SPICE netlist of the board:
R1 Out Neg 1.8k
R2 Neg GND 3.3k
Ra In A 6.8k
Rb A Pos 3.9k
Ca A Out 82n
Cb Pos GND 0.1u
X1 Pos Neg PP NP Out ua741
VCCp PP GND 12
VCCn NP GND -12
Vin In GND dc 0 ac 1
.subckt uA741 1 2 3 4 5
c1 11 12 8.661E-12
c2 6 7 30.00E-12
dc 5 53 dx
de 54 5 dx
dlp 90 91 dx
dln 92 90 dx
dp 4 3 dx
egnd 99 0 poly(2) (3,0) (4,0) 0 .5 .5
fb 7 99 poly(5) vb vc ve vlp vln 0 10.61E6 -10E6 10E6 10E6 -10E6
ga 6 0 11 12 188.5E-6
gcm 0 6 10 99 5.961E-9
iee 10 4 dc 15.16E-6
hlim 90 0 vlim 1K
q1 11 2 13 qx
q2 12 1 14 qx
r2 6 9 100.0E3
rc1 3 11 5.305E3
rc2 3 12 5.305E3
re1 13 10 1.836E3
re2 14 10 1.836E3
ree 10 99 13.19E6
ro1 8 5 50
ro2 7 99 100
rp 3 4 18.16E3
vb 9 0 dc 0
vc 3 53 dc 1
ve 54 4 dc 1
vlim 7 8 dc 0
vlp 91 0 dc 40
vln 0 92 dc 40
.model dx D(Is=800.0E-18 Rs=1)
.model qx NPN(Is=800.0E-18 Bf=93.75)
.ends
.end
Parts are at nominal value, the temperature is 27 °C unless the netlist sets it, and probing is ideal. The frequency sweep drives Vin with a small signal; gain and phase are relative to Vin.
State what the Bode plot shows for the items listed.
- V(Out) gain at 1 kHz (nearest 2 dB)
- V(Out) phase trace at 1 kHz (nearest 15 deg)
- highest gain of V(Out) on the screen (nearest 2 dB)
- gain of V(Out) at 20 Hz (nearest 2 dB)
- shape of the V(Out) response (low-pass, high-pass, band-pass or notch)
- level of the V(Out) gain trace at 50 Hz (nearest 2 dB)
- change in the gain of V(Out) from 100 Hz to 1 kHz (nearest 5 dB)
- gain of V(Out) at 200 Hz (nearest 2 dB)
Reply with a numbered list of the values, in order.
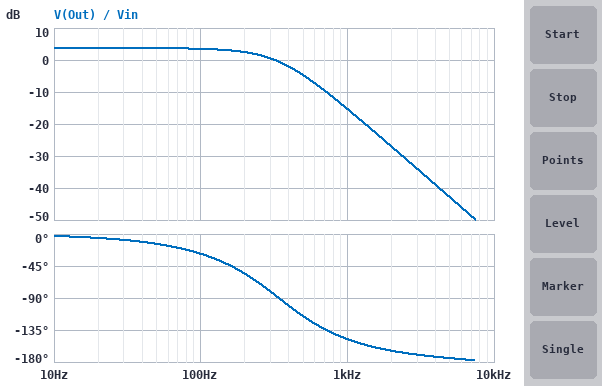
1. -16 dB
2. -150 deg
3. 4 dB
4. 4 dB
5. low-pass
6. 4 dB
7. -20 dB
8. 2 dB
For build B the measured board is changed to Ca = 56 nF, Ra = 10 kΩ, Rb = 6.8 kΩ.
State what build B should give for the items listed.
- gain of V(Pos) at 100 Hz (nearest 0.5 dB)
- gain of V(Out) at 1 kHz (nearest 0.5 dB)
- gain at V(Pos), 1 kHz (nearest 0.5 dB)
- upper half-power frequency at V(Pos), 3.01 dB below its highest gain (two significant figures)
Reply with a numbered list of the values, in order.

1. -1.5 dB
2. -20.5 dB
3. -24.5 dB
4. 140 Hz
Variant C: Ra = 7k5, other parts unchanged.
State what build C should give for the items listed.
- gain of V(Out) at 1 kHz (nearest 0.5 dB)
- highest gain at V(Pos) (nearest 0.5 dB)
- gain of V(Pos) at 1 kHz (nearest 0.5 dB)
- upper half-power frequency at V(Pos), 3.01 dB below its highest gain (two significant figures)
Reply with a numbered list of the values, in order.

1. -16.0 dB
2. 0 dB
3. -20.0 dB
4. 270 Hz
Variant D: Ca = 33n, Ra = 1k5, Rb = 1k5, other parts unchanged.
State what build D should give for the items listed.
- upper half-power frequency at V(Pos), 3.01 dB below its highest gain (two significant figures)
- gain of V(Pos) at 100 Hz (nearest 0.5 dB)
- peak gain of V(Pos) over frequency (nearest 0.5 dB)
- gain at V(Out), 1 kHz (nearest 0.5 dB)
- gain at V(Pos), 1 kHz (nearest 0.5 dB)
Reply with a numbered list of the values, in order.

1. 650 Hz
2. 0 dB
3. 0 dB
4. -1.5 dB
5. -5.5 dB
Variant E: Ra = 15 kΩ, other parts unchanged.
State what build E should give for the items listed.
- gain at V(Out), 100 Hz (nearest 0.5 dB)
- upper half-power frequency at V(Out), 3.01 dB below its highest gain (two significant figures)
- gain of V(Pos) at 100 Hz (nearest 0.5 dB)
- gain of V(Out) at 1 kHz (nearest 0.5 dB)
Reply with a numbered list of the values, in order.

1. 3.0 dB
2. 180 Hz
3. -1.0 dB
4. -22.0 dB
